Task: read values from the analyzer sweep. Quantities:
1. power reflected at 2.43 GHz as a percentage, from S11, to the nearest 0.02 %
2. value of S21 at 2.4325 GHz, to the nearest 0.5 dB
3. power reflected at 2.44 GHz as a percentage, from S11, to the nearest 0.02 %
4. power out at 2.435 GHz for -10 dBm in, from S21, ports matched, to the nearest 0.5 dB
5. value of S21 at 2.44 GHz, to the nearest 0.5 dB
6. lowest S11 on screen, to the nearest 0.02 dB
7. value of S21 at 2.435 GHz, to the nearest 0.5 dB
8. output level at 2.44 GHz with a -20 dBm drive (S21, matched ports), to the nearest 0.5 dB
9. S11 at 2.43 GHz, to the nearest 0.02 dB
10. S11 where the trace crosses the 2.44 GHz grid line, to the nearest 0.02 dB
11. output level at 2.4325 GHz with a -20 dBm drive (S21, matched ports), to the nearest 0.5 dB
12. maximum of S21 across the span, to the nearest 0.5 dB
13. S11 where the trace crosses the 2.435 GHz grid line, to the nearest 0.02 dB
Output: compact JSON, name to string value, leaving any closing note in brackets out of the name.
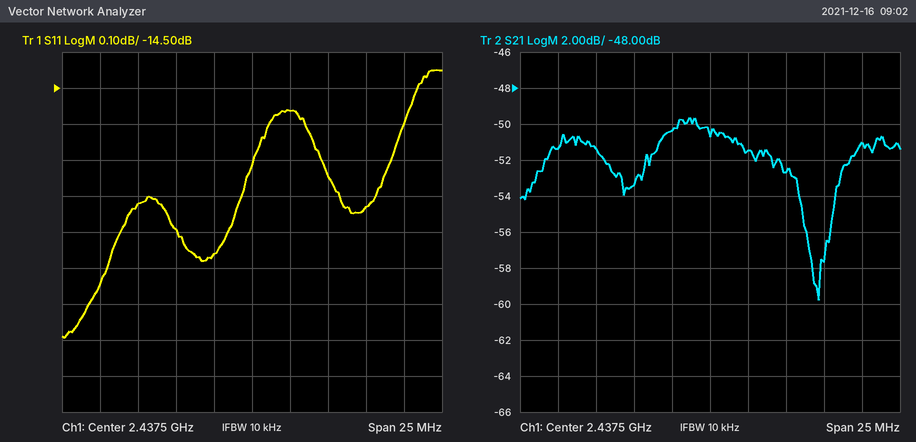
{"power reflected at 2.43 GHz as a percentage, from S11, to the nearest 0.02 %": "3.30 %", "value of S21 at 2.4325 GHz, to the nearest 0.5 dB": "-53.5 dB", "power reflected at 2.44 GHz as a percentage, from S11, to the nearest 0.02 %": "3.50 %", "power out at 2.435 GHz for -10 dBm in, from S21, ports matched, to the nearest 0.5 dB": "-60.5 dBm", "value of S21 at 2.44 GHz, to the nearest 0.5 dB": "-51.5 dB", "lowest S11 on screen, to the nearest 0.02 dB": "-15.20 dB", "value of S21 at 2.435 GHz, to the nearest 0.5 dB": "-50.5 dB", "output level at 2.44 GHz with a -20 dBm drive (S21, matched ports), to the nearest 0.5 dB": "-71.5 dBm", "S11 at 2.43 GHz, to the nearest 0.02 dB": "-14.82 dB", "S11 where the trace crosses the 2.44 GHz grid line, to the nearest 0.02 dB": "-14.56 dB", "output level at 2.4325 GHz with a -20 dBm drive (S21, matched ports), to the nearest 0.5 dB": "-73.5 dBm", "maximum of S21 across the span, to the nearest 0.5 dB": "-49.5 dB", "S11 where the trace crosses the 2.435 GHz grid line, to the nearest 0.02 dB": "-14.96 dB"}
